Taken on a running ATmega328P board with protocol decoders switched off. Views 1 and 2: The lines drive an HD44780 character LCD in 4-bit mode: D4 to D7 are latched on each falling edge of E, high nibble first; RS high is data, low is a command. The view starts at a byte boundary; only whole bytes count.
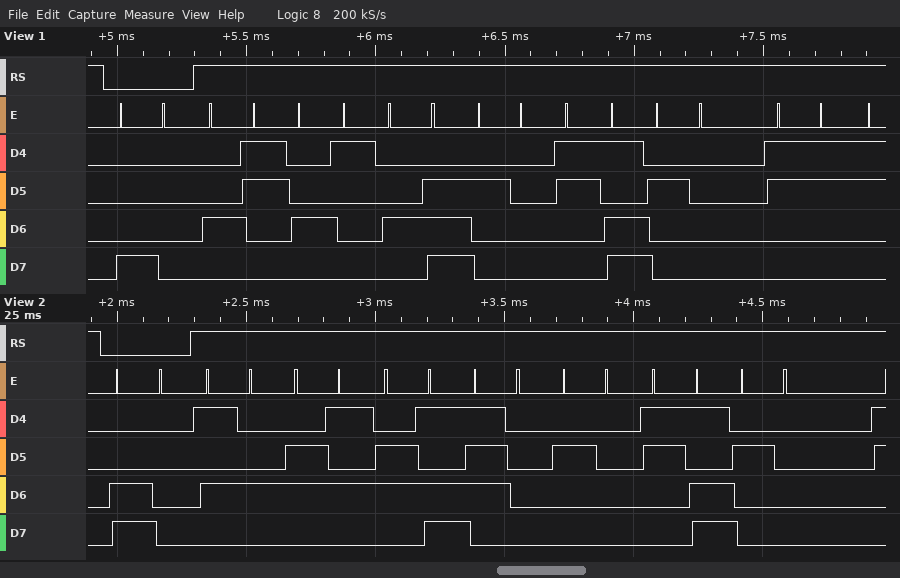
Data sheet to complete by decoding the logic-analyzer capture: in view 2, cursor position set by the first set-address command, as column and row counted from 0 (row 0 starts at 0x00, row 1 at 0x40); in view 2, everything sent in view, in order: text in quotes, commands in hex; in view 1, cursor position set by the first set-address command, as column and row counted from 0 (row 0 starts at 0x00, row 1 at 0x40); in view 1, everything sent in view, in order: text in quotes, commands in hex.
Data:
column 0, row 1
0xC0 "Temp = "
column 0, row 0
0x80 "CAN = 3"
